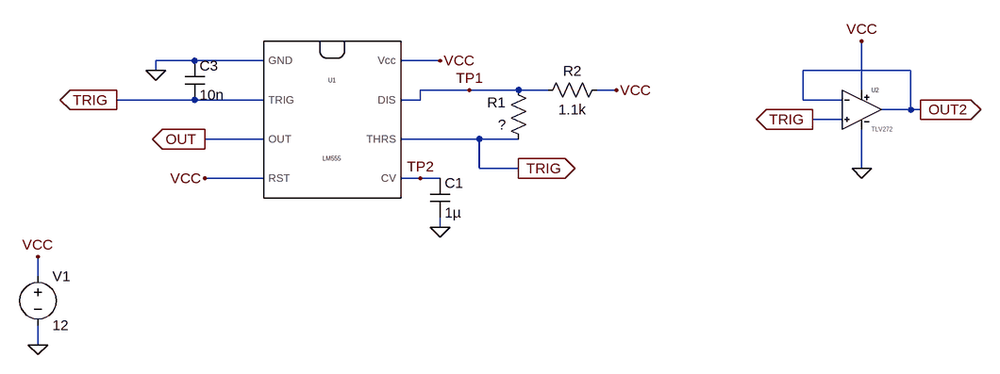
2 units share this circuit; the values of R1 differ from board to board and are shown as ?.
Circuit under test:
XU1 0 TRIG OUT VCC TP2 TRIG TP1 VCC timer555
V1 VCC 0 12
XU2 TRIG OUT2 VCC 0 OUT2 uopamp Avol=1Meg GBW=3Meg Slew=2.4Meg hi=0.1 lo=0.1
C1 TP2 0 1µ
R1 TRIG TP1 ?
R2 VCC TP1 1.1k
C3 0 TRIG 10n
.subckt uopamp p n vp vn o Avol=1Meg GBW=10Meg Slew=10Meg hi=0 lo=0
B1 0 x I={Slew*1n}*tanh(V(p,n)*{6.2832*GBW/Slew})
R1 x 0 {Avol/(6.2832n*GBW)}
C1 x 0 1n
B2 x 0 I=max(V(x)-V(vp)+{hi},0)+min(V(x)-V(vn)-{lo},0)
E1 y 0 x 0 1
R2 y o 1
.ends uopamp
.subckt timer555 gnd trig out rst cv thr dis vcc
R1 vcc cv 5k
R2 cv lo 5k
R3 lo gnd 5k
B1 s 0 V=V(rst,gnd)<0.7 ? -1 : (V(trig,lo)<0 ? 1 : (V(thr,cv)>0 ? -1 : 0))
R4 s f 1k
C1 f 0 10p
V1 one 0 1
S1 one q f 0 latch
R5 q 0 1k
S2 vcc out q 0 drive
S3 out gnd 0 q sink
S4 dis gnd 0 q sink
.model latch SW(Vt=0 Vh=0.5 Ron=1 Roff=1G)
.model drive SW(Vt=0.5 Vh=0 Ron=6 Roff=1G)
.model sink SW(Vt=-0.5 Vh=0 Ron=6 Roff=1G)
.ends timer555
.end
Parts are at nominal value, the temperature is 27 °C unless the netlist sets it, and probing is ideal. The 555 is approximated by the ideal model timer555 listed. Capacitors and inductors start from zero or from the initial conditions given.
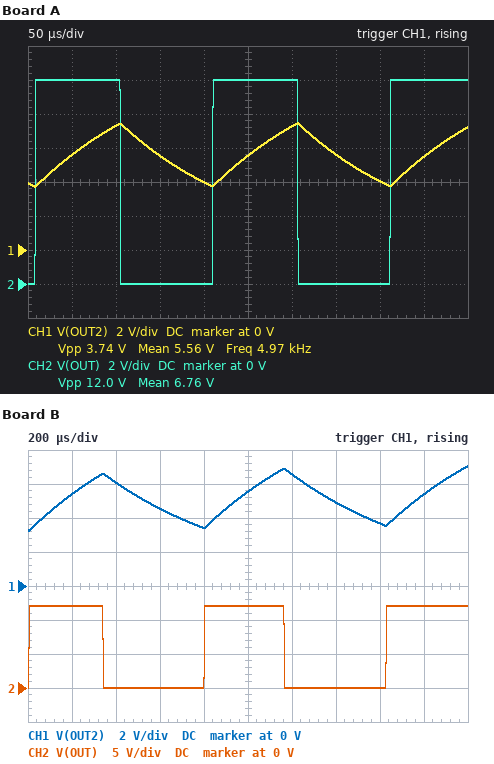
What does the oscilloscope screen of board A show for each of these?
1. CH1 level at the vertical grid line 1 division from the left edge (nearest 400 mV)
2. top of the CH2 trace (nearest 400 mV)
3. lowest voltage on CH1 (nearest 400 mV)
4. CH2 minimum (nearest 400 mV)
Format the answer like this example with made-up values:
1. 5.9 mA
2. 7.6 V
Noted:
1. 5.6 V
2. 12.0 V
3. 3.6 V
4. 0 V
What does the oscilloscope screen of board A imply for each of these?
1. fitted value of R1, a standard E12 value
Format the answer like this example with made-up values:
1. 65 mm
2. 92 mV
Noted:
1. 15 kΩ
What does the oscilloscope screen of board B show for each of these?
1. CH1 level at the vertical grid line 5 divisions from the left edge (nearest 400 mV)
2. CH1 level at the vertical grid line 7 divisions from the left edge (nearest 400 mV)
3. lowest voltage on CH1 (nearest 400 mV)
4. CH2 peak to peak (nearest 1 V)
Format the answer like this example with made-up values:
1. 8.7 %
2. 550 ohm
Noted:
1. 5.6 V
2. 4.8 V
3. 3.2 V
4. 12 V
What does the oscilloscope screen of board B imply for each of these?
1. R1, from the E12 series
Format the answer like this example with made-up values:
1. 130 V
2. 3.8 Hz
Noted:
1. 68 kΩ
